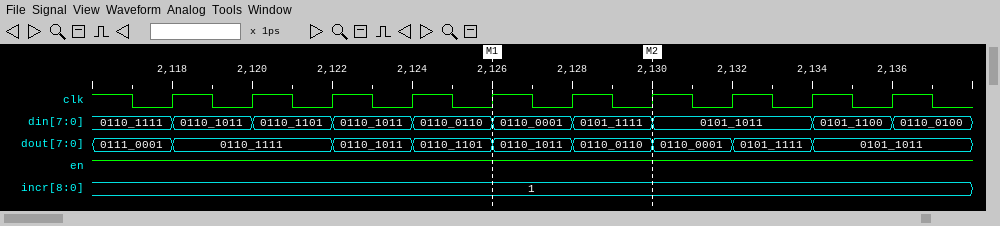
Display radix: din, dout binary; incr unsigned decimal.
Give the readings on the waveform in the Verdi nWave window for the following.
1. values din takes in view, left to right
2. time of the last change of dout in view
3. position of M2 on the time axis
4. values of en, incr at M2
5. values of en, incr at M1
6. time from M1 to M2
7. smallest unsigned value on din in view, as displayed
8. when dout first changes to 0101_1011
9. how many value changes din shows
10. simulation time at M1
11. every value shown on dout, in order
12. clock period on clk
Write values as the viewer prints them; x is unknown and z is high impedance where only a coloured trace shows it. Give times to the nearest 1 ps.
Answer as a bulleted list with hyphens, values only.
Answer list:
- 0110_1111, 0110_1011, 0110_1101, 0110_1011, 0110_0110, 0110_0001, 0101_1111, 0101_1011, 0101_1100, 0110_0100
- 2134 ps
- 2130 ps
- en=1, incr=1
- en=1, incr=1
- 4 ps
- 0101_1011
- 2134 ps
- 9
- 2126 ps
- 0111_0001, 0110_1111, 0110_1011, 0110_1101, 0110_1011, 0110_0110, 0110_0001, 0101_1111, 0101_1011
- 2 ps
